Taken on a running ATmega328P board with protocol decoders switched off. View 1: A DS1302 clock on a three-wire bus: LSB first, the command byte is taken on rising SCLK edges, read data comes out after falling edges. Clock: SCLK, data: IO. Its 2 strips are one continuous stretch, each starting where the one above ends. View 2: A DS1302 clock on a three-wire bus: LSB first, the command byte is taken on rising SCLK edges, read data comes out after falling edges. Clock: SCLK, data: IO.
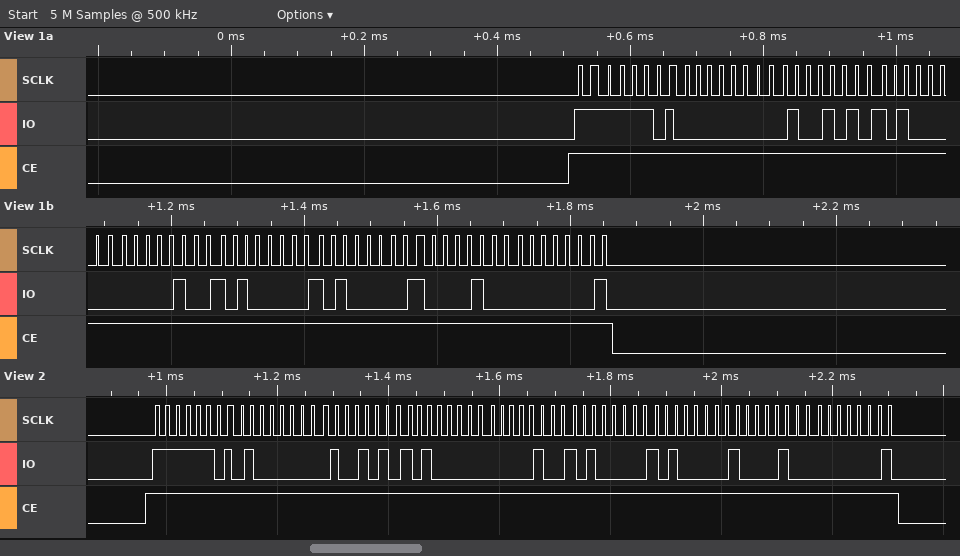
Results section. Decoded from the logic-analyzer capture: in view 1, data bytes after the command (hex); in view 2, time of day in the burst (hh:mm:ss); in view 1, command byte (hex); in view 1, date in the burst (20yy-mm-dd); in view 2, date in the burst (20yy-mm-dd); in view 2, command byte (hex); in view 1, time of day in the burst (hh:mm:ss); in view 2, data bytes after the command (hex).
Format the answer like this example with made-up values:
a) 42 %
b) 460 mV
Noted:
a) 00 52 05 20 05 05 21 80
b) 05:52:02
c) 0xBF
d) 2021-05-20
e) 2021-05-20
f) 0xBF
g) 05:52:00
h) 02 52 05 20 05 05 21 80
